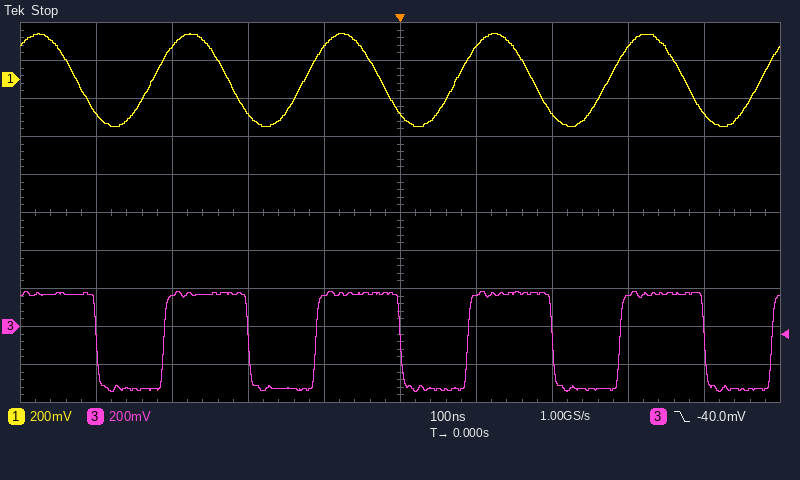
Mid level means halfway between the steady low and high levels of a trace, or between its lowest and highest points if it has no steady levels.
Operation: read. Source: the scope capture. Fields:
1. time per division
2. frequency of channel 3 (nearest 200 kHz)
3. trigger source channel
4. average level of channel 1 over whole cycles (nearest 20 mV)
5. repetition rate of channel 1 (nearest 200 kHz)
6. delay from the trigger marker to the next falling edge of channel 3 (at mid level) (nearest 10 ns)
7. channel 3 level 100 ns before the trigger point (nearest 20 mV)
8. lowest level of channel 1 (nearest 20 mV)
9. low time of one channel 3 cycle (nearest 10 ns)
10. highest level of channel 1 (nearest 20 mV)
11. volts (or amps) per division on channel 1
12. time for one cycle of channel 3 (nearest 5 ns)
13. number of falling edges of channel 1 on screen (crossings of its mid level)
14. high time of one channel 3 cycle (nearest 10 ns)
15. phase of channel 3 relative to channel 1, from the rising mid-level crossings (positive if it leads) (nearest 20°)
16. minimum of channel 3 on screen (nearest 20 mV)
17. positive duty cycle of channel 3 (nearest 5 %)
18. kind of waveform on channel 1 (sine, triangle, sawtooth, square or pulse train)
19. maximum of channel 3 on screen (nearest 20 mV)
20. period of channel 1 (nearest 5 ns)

100 ns
5.0 MHz
channel 3
0 mV
5.0 MHz
200 ns
160 mV
-240 mV
90 ns
240 mV
200 mV
200 ns
5
110 ns
-20°
-340 mV
55 %
sine
180 mV
200 ns
